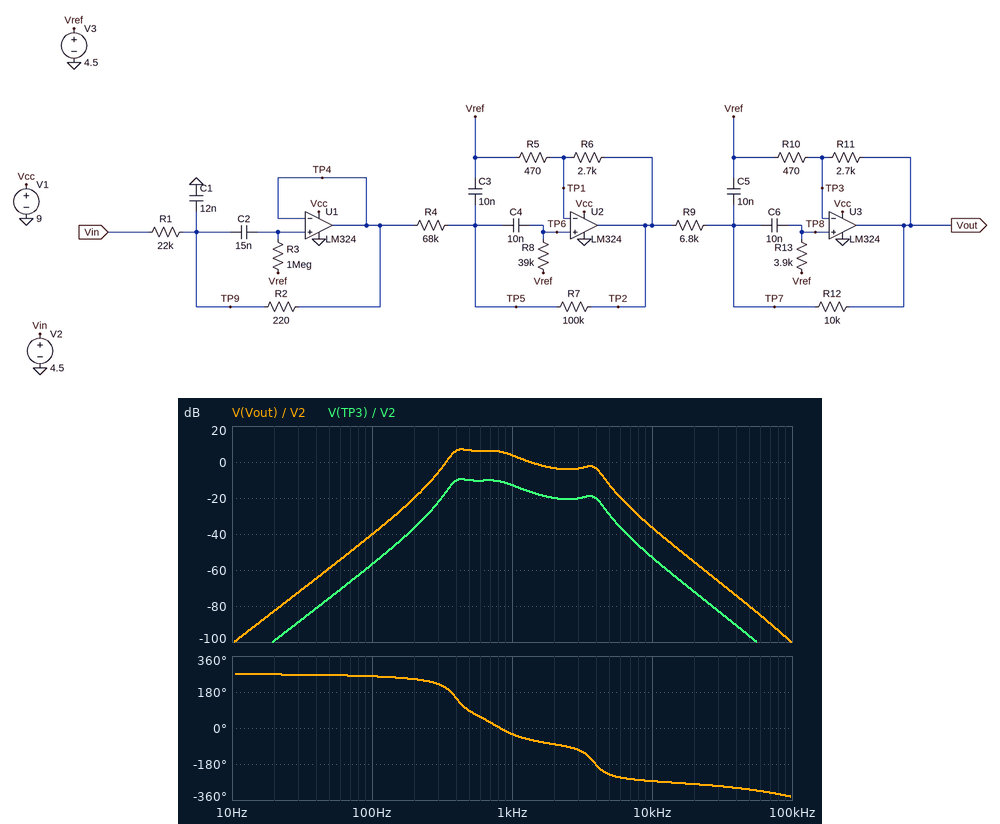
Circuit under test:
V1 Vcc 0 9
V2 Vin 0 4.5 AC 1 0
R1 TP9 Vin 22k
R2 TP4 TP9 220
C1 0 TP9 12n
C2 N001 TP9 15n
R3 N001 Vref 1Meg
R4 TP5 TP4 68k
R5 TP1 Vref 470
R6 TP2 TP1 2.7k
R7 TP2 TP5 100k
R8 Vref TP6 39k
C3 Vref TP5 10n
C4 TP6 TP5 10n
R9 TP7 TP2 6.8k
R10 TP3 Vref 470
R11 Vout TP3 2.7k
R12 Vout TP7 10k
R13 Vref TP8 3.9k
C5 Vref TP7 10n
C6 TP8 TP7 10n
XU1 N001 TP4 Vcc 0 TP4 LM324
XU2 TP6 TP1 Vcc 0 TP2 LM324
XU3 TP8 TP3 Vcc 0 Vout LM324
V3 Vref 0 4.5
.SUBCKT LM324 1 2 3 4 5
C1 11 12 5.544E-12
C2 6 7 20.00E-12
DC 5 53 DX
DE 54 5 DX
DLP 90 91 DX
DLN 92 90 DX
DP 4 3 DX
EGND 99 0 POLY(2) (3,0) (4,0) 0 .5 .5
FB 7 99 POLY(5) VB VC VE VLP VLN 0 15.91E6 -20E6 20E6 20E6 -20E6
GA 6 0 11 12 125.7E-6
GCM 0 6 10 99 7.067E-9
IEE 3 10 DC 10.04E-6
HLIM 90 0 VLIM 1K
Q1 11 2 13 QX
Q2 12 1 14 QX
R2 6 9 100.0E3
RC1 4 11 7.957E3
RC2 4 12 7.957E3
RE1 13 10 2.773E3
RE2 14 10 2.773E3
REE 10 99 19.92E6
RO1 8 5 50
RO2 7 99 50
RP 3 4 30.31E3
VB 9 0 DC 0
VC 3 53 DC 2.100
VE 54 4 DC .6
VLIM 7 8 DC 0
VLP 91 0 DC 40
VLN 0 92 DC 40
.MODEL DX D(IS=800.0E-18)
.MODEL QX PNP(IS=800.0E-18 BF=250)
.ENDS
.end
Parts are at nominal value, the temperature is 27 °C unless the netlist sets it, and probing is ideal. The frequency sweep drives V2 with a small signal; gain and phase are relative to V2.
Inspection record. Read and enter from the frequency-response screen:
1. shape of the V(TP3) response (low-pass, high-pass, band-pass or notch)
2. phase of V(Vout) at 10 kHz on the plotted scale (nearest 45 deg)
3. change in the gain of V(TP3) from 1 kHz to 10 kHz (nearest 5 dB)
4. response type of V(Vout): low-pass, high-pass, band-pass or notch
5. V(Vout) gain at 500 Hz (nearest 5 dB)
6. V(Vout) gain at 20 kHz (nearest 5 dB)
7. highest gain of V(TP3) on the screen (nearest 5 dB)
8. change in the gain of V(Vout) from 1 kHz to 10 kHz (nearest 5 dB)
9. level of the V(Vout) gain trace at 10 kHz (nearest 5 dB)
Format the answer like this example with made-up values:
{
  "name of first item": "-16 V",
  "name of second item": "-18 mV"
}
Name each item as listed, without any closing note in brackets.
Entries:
{
  "shape of the V(TP3) response": "band-pass",
  "phase of V(Vout) at 10 kHz on the plotted scale": "-270 deg",
  "change in the gain of V(TP3) from 1 kHz to 10 kHz": "-40 dB",
  "response type of V(Vout): low-pass, high-pass, band-pass or notch": "band-pass",
  "V(Vout) gain at 500 Hz": "5 dB",
  "V(Vout) gain at 20 kHz": "-55 dB",
  "highest gain of V(TP3) on the screen": "-10 dB",
  "change in the gain of V(Vout) from 1 kHz to 10 kHz": "-40 dB",
  "level of the V(Vout) gain trace at 10 kHz": "-35 dB"
}
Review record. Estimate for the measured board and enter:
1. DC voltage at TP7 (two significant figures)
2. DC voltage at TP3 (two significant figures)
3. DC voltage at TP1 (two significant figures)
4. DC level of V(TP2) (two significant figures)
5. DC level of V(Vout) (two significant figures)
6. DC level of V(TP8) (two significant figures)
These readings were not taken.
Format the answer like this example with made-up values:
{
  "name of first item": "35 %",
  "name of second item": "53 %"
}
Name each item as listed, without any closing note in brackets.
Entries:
{
  "DC voltage at TP7": "4.5 V",
  "DC voltage at TP3": "4.5 V",
  "DC voltage at TP1": "4.5 V",
  "DC level of V(TP2)": "4.5 V",
  "DC level of V(Vout)": "4.5 V",
  "DC level of V(TP8)": "4.5 V"
}
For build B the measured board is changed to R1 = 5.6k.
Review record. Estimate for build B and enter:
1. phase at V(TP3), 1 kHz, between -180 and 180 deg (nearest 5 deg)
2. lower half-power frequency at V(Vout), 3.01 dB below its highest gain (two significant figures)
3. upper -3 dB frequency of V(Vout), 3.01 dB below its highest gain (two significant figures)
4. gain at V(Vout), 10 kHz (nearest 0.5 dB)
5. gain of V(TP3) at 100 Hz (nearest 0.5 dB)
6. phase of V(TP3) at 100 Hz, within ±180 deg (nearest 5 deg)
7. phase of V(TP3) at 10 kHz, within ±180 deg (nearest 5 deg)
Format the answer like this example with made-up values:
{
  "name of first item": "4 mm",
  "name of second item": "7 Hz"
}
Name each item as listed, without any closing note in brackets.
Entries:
{
  "phase at V(TP3), 1 kHz, between -180 and 180 deg": "-5 deg",
  "lower half-power frequency at V(Vout), 3.01 dB below its highest gain": "360 Hz",
  "upper -3 dB frequency of V(Vout), 3.01 dB below its highest gain": "530 Hz",
  "gain at V(Vout), 10 kHz": "-24.5 dB",
  "gain of V(TP3) at 100 Hz": "-45.5 dB",
  "phase of V(TP3) at 100 Hz, within ±180 deg": "-115 deg",
  "phase of V(TP3) at 10 kHz, within ±180 deg": "105 deg"
}
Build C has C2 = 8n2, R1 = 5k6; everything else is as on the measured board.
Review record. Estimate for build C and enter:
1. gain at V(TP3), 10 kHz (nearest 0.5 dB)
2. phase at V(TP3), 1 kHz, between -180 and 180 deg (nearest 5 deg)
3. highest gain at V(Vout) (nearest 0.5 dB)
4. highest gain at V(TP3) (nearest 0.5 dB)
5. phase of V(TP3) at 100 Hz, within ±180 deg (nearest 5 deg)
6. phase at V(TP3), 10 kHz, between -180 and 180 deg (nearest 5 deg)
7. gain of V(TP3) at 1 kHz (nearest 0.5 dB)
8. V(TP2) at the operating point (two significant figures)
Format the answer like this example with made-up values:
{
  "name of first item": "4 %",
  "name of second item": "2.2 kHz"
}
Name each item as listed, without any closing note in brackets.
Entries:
{
  "gain at V(TP3), 10 kHz": "-41.0 dB",
  "phase at V(TP3), 1 kHz, between -180 and 180 deg": "5 deg",
  "highest gain at V(Vout)": "10.0 dB",
  "highest gain at V(TP3)": "-6.5 dB",
  "phase of V(TP3) at 100 Hz, within ±180 deg": "-105 deg",
  "phase at V(TP3), 10 kHz, between -180 and 180 deg": "105 deg",
  "gain of V(TP3) at 1 kHz": "-11.0 dB",
  "V(TP2) at the operating point": "4.5 V"
}
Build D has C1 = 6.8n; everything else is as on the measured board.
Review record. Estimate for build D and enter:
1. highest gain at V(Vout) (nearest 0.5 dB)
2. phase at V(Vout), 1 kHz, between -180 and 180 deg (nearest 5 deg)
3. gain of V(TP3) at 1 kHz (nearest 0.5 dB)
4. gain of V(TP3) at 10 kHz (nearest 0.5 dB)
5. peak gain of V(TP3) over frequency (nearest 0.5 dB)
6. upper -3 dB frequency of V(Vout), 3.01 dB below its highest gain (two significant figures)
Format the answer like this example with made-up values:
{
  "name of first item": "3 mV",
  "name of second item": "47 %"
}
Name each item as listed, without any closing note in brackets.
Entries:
{
  "highest gain at V(Vout)": "6.0 dB",
  "phase at V(Vout), 1 kHz, between -180 and 180 deg": "5 deg",
  "gain of V(TP3) at 1 kHz": "-11.0 dB",
  "gain of V(TP3) at 10 kHz": "-48.5 dB",
  "peak gain of V(TP3) over frequency": "-10.5 dB",
  "upper -3 dB frequency of V(Vout), 3.01 dB below its highest gain": "1.5 kHz"
}
